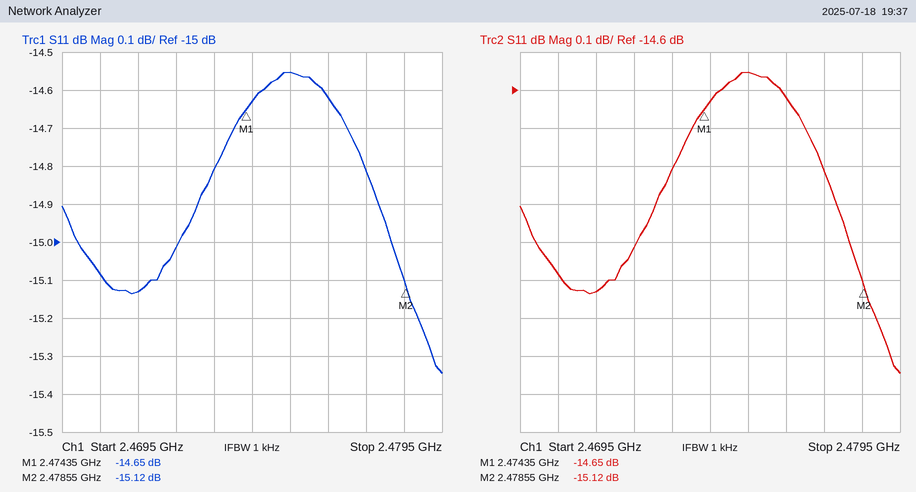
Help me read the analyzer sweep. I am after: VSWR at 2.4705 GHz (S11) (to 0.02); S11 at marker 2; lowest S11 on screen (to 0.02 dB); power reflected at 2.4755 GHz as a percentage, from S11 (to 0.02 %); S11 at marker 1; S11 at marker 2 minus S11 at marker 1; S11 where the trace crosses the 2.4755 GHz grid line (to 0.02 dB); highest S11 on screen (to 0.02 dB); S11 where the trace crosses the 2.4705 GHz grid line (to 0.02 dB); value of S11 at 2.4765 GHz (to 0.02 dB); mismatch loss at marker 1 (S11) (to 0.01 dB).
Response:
1.42
-15.12 dB
-15.34 dB
3.50 %
-14.65 dB
-0.47 dB
-14.56 dB
-14.56 dB
-15.08 dB
-14.62 dB
0.15 dB
